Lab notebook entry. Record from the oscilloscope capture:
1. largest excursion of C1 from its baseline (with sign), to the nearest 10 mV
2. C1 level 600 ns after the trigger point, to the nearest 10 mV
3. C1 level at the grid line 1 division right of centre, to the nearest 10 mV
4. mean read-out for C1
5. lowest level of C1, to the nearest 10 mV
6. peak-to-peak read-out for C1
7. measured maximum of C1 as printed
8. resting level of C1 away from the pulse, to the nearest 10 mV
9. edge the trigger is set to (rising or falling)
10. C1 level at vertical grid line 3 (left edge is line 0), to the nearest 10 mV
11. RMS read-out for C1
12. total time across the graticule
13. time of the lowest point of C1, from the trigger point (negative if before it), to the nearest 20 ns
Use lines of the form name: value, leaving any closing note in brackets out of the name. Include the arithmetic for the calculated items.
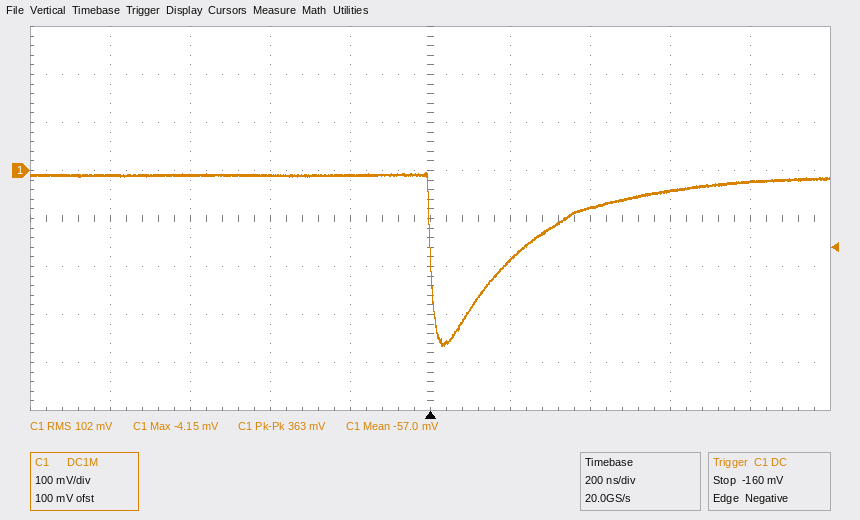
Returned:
largest excursion of C1 from its baseline (with sign), to the nearest 10 mV: -370 mV − (-10 mV) = -360 mV
C1 level 600 ns after the trigger point, to the nearest 10 mV: -40 mV
C1 level at the grid line 1 division right of centre, to the nearest 10 mV: -190 mV
mean read-out for C1: -57.0 mV
lowest level of C1, to the nearest 10 mV: -370 mV
peak-to-peak read-out for C1: 363 mV
measured maximum of C1 as printed: -4.15 mV
resting level of C1 away from the pulse, to the nearest 10 mV: -10 mV
edge the trigger is set to: falling
C1 level at vertical grid line 3 (left edge is line 0), to the nearest 10 mV: -10 mV
RMS read-out for C1: 102 mV
total time across the graticule: 2 µs
time of the lowest point of C1, from the trigger point (negative if before it), to the nearest 20 ns: +40 ns
